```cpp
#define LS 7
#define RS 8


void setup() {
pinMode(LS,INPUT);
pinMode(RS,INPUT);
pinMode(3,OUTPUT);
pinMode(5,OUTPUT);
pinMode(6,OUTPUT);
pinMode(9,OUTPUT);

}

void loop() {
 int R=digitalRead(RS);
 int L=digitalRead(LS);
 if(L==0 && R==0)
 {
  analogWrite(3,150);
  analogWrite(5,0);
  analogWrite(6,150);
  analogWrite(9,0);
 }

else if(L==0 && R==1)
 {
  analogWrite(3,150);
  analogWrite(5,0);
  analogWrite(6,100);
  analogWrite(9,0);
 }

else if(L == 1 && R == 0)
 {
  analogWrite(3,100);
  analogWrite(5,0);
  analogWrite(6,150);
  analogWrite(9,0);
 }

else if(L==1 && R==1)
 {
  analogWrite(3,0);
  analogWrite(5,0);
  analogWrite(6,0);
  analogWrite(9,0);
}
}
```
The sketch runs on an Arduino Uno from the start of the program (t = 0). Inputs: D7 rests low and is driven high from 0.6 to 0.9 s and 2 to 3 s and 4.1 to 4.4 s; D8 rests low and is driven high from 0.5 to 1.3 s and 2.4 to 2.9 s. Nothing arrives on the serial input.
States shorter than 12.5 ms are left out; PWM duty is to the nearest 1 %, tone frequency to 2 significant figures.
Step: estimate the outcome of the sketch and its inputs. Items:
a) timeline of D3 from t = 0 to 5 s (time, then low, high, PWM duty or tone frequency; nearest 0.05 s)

0 s PWM 59 %; 0.6 s low; 0.9 s PWM 59 %; 2 s PWM 39 %; 2.4 s low; 2.9 s PWM 39 %; 3 s PWM 59 %; 4.1 s PWM 39 %; 4.4 s PWM 59 %
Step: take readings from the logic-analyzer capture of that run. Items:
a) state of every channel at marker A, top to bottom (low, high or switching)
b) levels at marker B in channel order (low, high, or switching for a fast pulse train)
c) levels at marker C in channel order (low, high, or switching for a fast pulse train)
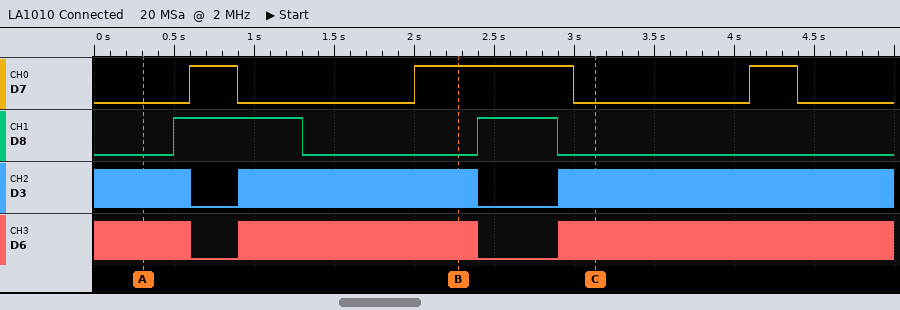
D7 low, D8 low, D3 switching, D6 switching
D7 high, D8 low, D3 switching, D6 switching
D7 low, D8 low, D3 switching, D6 switching
